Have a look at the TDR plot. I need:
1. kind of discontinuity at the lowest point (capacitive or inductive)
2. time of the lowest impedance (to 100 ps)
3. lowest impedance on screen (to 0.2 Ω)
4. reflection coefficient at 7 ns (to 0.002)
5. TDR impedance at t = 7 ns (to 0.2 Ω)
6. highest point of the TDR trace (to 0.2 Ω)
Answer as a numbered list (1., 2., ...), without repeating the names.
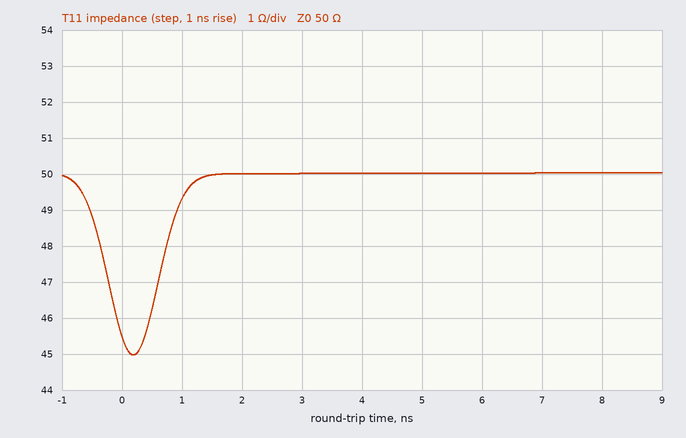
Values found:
1. capacitive
2. 200 ps
3. 45.0 Ω
4. 0.000
5. 50.0 Ω
6. 50.0 Ω
